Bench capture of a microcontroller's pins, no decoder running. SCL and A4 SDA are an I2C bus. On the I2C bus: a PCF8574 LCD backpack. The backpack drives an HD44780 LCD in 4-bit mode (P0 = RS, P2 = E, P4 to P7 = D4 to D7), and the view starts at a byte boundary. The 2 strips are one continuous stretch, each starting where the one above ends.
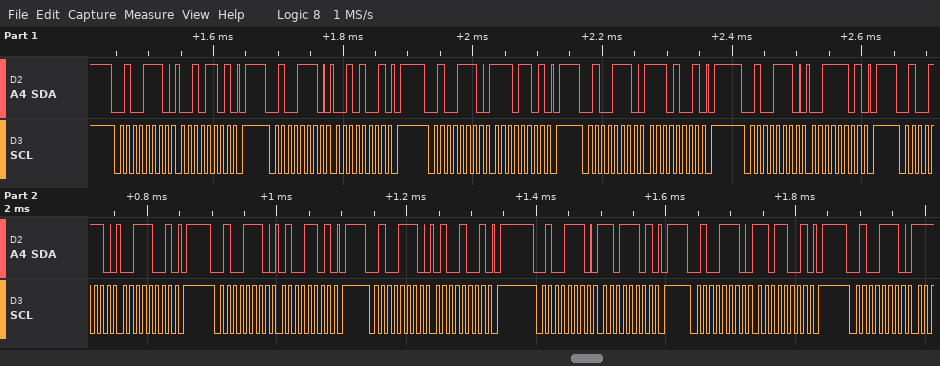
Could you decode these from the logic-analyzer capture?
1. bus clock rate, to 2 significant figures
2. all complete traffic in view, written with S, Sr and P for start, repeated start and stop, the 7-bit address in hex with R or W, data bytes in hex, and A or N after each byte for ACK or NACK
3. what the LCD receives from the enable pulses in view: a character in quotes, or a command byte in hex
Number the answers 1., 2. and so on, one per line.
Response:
1. 100 kHz
2. S 27W A 2D A P S 27W A 29 A P S 27W A ED A P S 27W A E9 A P S 27W A 3D A P S 27W A 39 A P S 27W A 4D A P S 27W A 49 A P S 27W A DD A P S 27W A D9 A P S 27W A
3. '.' '4'
